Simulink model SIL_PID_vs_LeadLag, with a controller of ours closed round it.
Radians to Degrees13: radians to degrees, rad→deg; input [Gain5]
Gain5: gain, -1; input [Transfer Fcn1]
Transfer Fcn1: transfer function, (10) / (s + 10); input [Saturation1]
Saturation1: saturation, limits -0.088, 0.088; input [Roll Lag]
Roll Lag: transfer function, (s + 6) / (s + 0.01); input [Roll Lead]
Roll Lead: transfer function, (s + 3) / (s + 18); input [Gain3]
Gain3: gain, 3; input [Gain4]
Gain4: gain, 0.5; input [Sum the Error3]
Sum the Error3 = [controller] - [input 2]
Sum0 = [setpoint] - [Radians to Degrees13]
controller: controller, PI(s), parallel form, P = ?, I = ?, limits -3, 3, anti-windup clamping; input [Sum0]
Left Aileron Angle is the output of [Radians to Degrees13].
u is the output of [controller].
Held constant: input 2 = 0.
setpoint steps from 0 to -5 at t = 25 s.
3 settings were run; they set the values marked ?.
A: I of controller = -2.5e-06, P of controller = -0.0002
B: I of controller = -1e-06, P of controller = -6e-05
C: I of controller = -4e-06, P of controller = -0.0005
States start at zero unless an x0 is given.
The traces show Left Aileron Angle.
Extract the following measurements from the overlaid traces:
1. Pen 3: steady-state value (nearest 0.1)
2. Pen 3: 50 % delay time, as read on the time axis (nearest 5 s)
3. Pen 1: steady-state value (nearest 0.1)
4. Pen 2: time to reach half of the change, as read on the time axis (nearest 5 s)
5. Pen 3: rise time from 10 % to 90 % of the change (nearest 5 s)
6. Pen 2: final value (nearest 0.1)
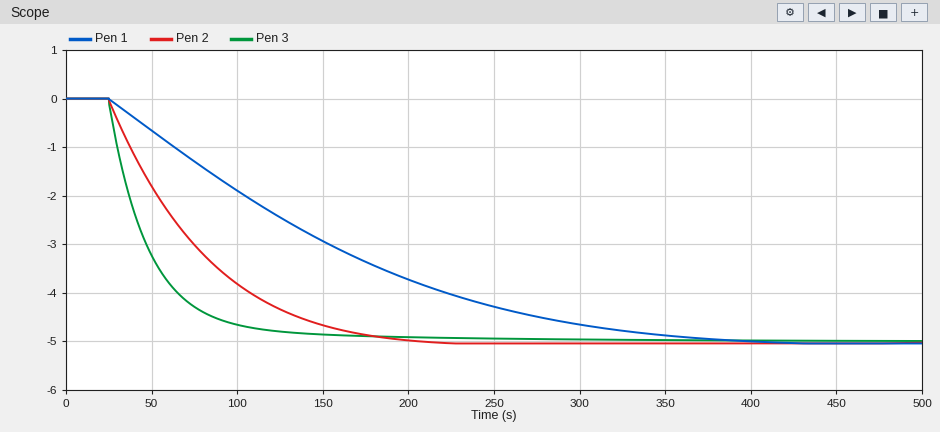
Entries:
-5.0
40 s
-5.0
65 s
60 s
-5.0
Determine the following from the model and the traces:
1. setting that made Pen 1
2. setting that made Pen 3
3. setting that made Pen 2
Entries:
B
C
A
